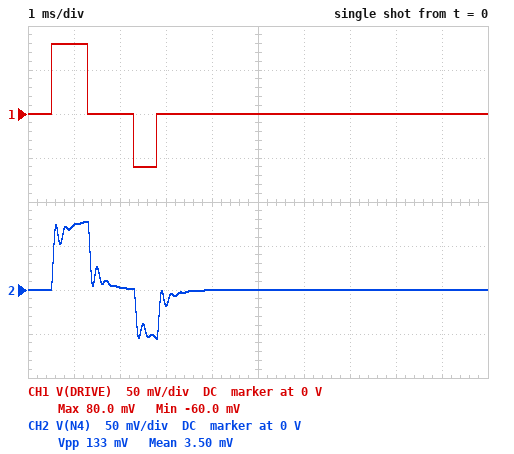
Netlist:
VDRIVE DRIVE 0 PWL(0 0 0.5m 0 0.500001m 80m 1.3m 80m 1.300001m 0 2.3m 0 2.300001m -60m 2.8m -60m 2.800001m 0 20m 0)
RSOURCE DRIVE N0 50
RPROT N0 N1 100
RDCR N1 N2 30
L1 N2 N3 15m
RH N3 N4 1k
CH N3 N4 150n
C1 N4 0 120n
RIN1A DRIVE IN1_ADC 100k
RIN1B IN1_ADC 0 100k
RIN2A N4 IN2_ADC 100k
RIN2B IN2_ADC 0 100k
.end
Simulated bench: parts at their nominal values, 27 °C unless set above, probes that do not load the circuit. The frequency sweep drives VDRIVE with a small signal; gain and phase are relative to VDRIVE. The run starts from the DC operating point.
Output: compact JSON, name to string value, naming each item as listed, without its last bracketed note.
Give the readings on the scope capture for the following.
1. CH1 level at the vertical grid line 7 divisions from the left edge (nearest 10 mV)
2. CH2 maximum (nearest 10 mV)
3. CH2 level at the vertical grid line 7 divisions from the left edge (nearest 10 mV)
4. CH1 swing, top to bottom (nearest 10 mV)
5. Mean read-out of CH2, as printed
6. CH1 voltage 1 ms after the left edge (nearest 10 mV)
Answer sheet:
{"CH1 level at the vertical grid line 7 divisions from the left edge": "0 V", "CH2 maximum": "80 mV", "CH2 level at the vertical grid line 7 divisions from the left edge": "0 V", "CH1 swing, top to bottom": "140 mV", "Mean read-out of CH2, as printed": "3.50 mV", "CH1 voltage 1 ms after the left edge": "80 mV"}
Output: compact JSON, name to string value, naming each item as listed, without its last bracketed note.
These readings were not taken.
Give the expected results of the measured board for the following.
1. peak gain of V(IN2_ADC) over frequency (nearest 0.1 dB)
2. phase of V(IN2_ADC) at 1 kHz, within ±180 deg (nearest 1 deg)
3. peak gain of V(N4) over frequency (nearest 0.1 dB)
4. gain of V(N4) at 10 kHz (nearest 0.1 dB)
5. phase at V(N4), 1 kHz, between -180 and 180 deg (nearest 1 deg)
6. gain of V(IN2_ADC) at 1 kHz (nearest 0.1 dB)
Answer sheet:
{"peak gain of V(IN2_ADC) over frequency": "-4.4 dB", "phase of V(IN2_ADC) at 1 kHz, within ±180 deg": "-22 deg", "peak gain of V(N4) over frequency": "1.6 dB", "gain of V(N4) at 10 kHz": "-14.8 dB", "phase at V(N4), 1 kHz, between -180 and 180 deg": "-22 deg", "gain of V(IN2_ADC) at 1 kHz": "-9.0 dB"}
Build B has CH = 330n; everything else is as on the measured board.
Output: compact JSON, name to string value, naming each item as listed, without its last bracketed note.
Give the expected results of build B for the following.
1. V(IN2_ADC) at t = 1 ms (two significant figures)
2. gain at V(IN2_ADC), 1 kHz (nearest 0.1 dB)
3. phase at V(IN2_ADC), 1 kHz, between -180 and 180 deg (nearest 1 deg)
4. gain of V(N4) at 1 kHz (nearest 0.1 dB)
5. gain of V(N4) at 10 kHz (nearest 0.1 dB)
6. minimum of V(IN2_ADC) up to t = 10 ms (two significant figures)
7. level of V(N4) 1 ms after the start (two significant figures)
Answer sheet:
{"V(IN2_ADC) at t = 1 ms": "35 mV", "gain at V(IN2_ADC), 1 kHz": "-8.0 dB", "phase at V(IN2_ADC), 1 kHz, between -180 and 180 deg": "-13 deg", "gain of V(N4) at 1 kHz": "-2.0 dB", "gain of V(N4) at 10 kHz": "-15.4 dB", "minimum of V(IN2_ADC) up to t = 10 ms": "-33 mV", "level of V(N4) 1 ms after the start": "70 mV"}
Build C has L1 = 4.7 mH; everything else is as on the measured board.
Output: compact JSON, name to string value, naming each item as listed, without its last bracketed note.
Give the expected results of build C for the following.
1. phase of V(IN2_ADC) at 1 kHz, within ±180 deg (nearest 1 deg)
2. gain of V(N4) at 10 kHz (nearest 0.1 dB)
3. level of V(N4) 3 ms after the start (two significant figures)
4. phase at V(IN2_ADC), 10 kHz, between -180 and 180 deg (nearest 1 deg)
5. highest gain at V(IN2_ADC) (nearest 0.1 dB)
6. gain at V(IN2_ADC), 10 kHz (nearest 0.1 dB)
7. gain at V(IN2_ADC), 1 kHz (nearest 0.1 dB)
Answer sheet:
{"phase of V(IN2_ADC) at 1 kHz, within ±180 deg": "-21 deg", "gain of V(N4) at 10 kHz": "-3.6 dB", "level of V(N4) 3 ms after the start": "-11 mV", "phase at V(IN2_ADC), 10 kHz, between -180 and 180 deg": "-107 deg", "highest gain at V(IN2_ADC)": "-6.1 dB", "gain at V(IN2_ADC), 10 kHz": "-9.6 dB", "gain at V(IN2_ADC), 1 kHz": "-9.3 dB"}
